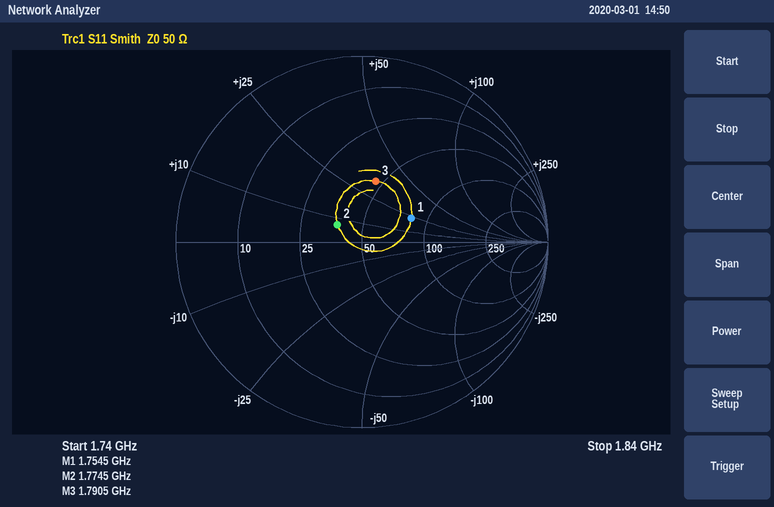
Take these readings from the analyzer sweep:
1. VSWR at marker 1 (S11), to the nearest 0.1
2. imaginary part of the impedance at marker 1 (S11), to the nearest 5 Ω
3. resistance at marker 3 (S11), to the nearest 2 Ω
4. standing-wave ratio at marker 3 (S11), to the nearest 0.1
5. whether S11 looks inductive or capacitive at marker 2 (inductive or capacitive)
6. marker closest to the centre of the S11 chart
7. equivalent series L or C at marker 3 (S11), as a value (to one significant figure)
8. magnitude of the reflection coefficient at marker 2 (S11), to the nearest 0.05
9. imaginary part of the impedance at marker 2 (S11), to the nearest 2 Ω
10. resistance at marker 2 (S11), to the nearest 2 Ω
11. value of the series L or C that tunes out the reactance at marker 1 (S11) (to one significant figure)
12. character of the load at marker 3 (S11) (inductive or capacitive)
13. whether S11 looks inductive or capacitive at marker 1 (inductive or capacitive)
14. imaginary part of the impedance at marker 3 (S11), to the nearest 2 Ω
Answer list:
1.8
+25 Ω
46 Ω
2.0
inductive
marker 2
3 nH
0.15
+8 Ω
38 Ω
4 pF
inductive
inductive
+34 Ω
